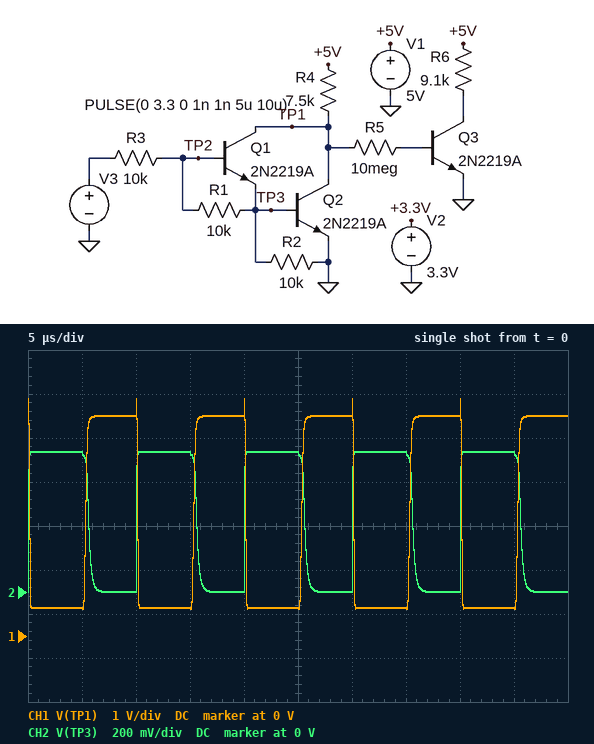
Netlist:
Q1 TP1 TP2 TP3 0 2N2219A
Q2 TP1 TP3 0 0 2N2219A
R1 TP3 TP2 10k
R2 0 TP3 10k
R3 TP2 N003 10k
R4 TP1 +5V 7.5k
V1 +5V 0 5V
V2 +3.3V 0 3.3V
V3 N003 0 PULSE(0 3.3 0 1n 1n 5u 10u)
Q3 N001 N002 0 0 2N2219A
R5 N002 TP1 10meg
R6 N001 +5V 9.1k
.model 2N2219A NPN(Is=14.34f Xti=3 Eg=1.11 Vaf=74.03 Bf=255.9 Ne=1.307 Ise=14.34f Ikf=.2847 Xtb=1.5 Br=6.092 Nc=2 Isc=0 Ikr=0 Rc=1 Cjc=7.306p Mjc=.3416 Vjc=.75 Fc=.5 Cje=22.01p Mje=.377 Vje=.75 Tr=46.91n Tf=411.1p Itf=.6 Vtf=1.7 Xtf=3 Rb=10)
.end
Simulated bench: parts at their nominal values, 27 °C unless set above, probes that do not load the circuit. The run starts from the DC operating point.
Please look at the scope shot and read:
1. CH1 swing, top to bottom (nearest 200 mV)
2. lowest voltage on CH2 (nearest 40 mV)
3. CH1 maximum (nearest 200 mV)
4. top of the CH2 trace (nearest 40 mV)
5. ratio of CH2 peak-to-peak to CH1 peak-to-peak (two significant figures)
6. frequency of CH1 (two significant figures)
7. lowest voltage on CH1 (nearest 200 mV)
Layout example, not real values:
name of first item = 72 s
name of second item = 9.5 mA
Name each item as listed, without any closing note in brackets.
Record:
CH1 swing, top to bottom = 4.8 V
lowest voltage on CH2 = 0 V
CH1 maximum = 5.4 V
top of the CH2 trace = 640 mV
ratio of CH2 peak-to-peak to CH1 peak-to-peak = 0.13
frequency of CH1 = 100 kHz
lowest voltage on CH1 = 600 mV
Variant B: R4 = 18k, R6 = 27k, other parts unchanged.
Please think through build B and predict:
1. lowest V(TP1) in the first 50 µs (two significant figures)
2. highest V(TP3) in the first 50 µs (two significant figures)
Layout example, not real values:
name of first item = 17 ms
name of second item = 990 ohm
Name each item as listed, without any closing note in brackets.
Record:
lowest V(TP1) in the first 50 µs = 580 mV
highest V(TP3) in the first 50 µs = 620 mV
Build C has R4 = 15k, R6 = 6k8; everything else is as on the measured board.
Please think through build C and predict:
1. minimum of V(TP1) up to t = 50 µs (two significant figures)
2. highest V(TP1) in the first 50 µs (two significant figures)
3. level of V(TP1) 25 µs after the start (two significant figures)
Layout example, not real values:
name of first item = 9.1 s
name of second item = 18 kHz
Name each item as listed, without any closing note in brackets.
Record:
minimum of V(TP1) up to t = 50 µs = 590 mV
highest V(TP1) in the first 50 µs = 5.5 V
level of V(TP1) 25 µs after the start = 620 mV
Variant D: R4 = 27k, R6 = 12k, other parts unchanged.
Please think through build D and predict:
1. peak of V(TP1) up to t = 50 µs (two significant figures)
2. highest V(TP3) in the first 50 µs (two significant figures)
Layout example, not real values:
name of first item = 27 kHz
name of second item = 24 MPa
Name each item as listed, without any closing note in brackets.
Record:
peak of V(TP1) up to t = 50 µs = 5.6 V
highest V(TP3) in the first 50 µs = 620 mV
